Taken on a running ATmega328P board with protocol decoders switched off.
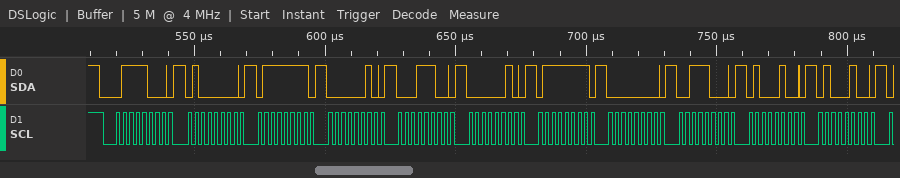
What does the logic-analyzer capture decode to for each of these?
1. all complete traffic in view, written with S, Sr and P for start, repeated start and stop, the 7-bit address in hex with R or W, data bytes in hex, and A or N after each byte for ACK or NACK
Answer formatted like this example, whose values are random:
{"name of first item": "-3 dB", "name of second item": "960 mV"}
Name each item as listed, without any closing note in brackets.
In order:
{"all complete traffic in view, written with S, Sr and P for start, repeated start and stop, the 7-bit address in hex with R or W, data bytes in hex, and A or N after each byte for ACK or NACK": "S 3CW A 40 A 7F A 02 A 1C A 02 A 7F A 00 A 38 A 44 A 44 A"}
